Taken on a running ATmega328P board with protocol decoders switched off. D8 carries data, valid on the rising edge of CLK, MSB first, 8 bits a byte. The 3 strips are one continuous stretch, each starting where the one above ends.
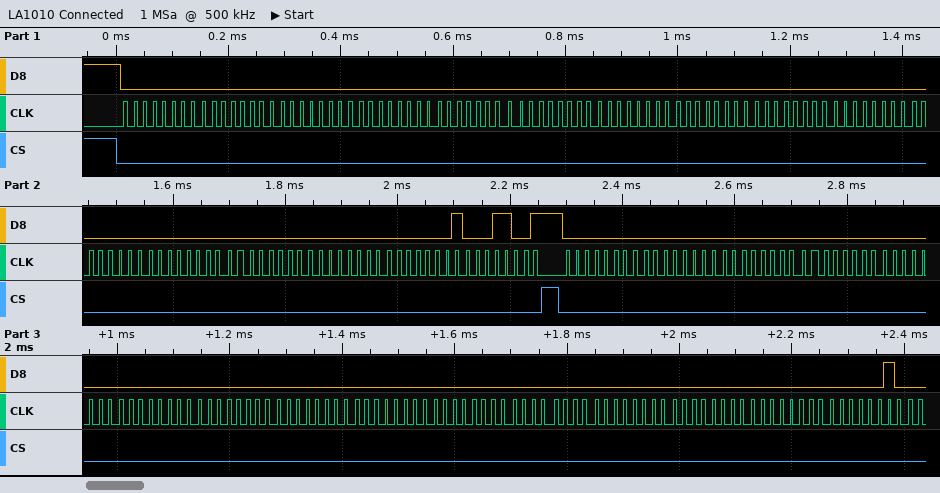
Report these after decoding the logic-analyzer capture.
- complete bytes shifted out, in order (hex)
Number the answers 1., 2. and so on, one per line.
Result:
1. 00 00 00 00 00 00 00 00 00 00 00 00 00 00 01 19 00 00 00 00 00 00 00 00 00 00 00 00 00 00 02
